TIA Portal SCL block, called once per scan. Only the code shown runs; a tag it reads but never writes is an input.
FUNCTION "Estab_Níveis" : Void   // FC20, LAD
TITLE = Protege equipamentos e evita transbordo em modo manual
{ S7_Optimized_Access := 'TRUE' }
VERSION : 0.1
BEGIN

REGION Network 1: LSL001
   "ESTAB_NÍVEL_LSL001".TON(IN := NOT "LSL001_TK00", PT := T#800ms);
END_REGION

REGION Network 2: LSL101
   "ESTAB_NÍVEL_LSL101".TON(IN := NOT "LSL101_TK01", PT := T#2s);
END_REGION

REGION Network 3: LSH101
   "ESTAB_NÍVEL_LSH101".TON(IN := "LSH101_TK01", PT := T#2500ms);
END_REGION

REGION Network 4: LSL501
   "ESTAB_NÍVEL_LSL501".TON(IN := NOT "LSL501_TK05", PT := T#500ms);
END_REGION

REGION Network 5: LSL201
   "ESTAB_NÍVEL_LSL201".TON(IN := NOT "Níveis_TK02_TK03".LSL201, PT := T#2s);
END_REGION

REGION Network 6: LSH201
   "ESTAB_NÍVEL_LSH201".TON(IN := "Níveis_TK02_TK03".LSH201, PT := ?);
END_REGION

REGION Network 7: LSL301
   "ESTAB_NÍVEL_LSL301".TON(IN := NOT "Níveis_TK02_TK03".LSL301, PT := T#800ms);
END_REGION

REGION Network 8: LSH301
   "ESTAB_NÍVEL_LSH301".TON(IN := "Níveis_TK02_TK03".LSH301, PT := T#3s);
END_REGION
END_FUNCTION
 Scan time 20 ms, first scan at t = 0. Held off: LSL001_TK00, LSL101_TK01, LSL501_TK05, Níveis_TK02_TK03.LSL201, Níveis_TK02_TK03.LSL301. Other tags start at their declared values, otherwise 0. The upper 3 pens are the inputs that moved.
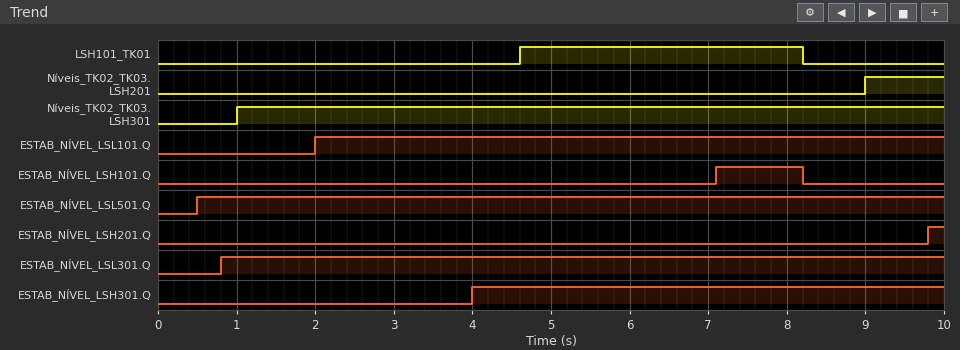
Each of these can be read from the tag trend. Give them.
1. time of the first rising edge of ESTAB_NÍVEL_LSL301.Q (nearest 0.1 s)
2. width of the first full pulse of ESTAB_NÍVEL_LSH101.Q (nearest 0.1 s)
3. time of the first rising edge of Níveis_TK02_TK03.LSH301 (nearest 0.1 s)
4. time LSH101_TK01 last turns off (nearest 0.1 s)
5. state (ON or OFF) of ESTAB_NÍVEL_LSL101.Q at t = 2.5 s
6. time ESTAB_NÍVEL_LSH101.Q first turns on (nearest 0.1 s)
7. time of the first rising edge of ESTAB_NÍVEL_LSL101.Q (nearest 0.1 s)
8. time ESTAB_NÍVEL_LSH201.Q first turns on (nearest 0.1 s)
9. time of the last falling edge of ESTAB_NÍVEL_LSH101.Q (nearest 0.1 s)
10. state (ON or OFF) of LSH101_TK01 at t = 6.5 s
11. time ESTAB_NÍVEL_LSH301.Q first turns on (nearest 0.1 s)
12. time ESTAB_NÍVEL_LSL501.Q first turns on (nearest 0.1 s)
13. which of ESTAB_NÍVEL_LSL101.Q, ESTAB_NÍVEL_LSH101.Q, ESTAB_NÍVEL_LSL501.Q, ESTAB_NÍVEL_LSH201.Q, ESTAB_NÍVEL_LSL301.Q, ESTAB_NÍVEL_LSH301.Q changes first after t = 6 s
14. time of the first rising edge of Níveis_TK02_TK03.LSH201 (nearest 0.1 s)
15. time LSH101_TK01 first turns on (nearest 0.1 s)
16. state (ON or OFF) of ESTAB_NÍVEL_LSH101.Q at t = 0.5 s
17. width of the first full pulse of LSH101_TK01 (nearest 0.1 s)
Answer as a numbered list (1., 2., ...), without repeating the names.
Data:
1. 0.8 s
2. 1.1 s
3. 1.0 s
4. 8.2 s
5. ON
6. 7.1 s
7. 2.0 s
8. 9.8 s
9. 8.2 s
10. ON
11. 4.0 s
12. 0.5 s
13. ESTAB_NÍVEL_LSH101.Q
14. 9.0 s
15. 4.6 s
16. OFF
17. 3.6 s
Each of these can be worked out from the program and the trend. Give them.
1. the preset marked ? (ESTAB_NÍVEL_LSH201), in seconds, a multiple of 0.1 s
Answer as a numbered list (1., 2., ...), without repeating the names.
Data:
1. 0.8 s
